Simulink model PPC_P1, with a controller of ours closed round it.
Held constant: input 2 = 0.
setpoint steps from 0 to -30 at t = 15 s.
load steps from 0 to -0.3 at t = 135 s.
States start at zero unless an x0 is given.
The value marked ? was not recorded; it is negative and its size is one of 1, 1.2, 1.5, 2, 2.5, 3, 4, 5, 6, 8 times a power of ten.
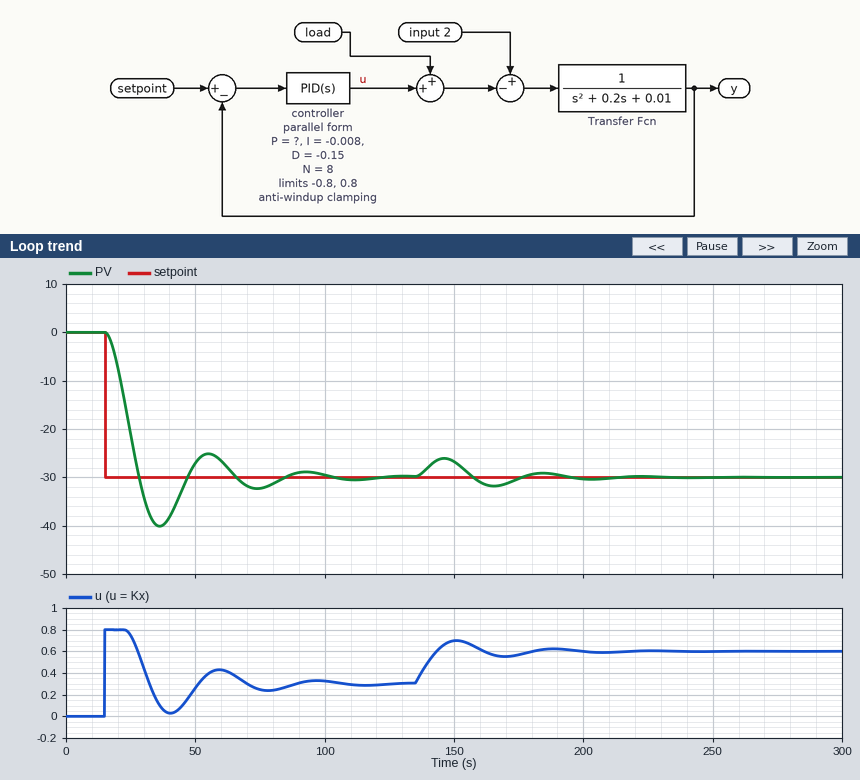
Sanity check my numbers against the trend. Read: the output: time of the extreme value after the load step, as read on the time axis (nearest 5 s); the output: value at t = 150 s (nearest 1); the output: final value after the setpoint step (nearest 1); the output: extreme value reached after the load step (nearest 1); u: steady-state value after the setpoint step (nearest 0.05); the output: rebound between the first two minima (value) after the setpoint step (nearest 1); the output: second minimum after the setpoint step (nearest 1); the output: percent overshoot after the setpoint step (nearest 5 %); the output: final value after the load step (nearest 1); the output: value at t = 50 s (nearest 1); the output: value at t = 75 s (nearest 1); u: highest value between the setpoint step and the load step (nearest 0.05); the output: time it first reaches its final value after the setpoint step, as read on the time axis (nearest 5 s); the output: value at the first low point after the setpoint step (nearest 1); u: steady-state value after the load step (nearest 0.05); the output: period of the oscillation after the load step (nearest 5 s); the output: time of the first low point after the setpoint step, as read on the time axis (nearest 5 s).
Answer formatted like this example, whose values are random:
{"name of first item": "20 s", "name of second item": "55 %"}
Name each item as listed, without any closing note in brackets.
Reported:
{"the output: time of the extreme value after the load step, as read on the time axis": "145 s", "the output: value at t = 150 s": "-27", "the output: final value after the setpoint step": "-30", "the output: extreme value reached after the load step": "-26", "u: steady-state value after the setpoint step": "0.30", "the output: rebound between the first two minima (value) after the setpoint step": "-25", "the output: second minimum after the setpoint step": "-32", "the output: percent overshoot after the setpoint step": "35 %", "the output: final value after the load step": "-30", "the output: value at t = 50 s": "-27", "the output: value at t = 75 s": "-32", "u: highest value between the setpoint step and the load step": "0.80", "the output: time it first reaches its final value after the setpoint step, as read on the time axis": "30 s", "the output: value at the first low point after the setpoint step": "-40", "u: steady-state value after the load step": "0.60", "the output: period of the oscillation after the load step": "40 s", "the output: time of the first low point after the setpoint step, as read on the time axis": "35 s"}
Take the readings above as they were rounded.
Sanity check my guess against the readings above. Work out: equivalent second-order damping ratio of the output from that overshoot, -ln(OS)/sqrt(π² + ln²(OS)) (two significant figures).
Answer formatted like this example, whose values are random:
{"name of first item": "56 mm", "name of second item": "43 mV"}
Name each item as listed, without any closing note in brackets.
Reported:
{"equivalent second-order damping ratio of the output from that overshoot, -ln(OS)/sqrt(π² + ln²(OS))": "0.32"}
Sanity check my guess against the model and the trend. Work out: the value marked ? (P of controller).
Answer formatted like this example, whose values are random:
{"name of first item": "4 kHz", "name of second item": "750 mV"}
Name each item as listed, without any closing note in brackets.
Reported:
{"the value marked ?": "-0.04"}
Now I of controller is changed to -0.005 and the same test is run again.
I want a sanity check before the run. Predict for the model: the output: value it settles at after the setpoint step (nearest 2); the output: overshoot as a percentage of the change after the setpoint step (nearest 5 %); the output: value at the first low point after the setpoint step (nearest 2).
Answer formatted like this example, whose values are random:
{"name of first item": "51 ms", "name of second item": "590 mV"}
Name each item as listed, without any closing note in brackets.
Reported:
{"the output: value it settles at after the setpoint step": "-30", "the output: overshoot as a percentage of the change after the setpoint step": "25 %", "the output: value at the first low point after the setpoint step": "-38"}
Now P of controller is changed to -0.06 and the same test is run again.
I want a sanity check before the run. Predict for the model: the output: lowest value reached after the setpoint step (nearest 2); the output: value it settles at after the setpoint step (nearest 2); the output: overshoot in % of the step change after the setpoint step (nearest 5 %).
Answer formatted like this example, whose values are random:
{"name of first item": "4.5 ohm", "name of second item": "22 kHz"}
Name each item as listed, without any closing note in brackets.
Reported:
{"the output: lowest value reached after the setpoint step": "-34", "the output: value it settles at after the setpoint step": "-30", "the output: overshoot in % of the step change after the setpoint step": "15 %"}
